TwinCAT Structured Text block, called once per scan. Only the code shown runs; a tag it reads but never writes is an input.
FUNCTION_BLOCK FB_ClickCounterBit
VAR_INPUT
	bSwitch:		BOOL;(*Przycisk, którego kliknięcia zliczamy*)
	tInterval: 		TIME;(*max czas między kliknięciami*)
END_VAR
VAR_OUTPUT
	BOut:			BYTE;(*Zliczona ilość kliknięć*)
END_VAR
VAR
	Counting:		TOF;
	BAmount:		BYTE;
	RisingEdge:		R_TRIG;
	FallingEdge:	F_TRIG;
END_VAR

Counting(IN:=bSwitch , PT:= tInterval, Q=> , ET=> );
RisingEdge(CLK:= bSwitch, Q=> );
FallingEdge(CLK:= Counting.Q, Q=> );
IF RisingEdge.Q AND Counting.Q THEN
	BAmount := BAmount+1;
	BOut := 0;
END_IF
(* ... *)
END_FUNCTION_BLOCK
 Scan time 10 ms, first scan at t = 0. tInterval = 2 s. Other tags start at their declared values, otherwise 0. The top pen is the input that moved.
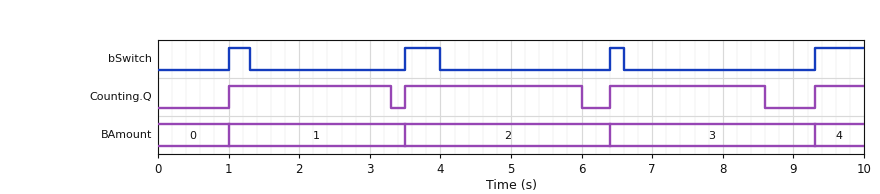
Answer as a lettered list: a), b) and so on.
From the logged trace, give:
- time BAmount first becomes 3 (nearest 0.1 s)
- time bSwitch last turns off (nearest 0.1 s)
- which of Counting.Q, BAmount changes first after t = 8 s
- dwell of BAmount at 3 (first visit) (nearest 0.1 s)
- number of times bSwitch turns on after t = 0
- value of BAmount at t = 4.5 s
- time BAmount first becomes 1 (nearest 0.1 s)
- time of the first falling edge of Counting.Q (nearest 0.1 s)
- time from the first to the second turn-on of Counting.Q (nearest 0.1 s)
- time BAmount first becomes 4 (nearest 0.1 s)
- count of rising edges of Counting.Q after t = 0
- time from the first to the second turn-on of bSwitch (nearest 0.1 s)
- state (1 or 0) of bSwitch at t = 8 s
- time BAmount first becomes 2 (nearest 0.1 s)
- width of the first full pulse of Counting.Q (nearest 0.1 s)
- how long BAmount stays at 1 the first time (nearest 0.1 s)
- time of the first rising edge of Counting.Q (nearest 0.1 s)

a) 6.4 s
b) 6.6 s
c) Counting.Q
d) 2.9 s
e) 4
f) 2
g) 1.0 s
h) 3.3 s
i) 2.5 s
j) 9.3 s
k) 4
l) 2.5 s
m) 0
n) 3.5 s
o) 2.3 s
p) 2.5 s
q) 1.0 s
